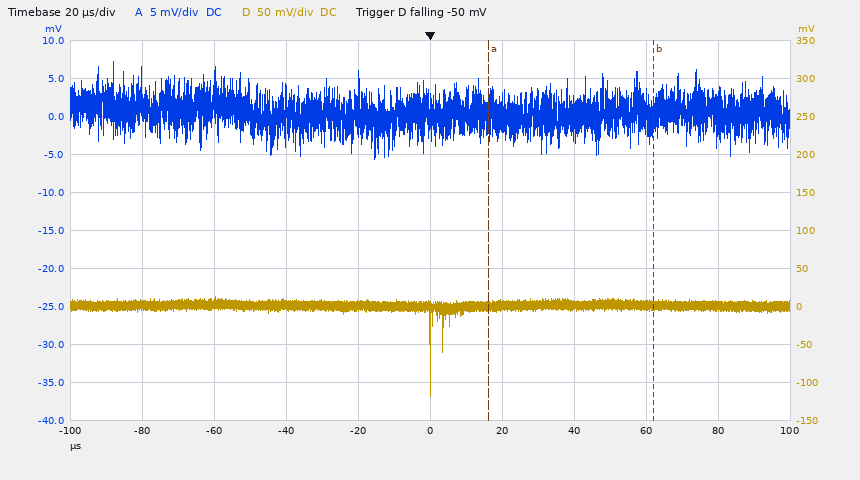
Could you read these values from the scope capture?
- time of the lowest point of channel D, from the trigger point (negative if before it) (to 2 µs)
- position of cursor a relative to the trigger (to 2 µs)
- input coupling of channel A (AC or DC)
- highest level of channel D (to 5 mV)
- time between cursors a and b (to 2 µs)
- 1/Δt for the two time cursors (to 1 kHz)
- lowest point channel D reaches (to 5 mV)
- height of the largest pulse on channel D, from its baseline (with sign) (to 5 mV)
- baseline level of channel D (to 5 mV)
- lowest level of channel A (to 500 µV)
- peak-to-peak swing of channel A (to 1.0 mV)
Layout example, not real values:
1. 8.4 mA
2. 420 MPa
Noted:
1. 0 µs
2. +16 µs
3. DC
4. 15 mV
5. 46 µs
6. 22 kHz
7. -120 mV
8. -120 mV
9. 0 mV
10. -5.5 mV
11. 13.0 mV
